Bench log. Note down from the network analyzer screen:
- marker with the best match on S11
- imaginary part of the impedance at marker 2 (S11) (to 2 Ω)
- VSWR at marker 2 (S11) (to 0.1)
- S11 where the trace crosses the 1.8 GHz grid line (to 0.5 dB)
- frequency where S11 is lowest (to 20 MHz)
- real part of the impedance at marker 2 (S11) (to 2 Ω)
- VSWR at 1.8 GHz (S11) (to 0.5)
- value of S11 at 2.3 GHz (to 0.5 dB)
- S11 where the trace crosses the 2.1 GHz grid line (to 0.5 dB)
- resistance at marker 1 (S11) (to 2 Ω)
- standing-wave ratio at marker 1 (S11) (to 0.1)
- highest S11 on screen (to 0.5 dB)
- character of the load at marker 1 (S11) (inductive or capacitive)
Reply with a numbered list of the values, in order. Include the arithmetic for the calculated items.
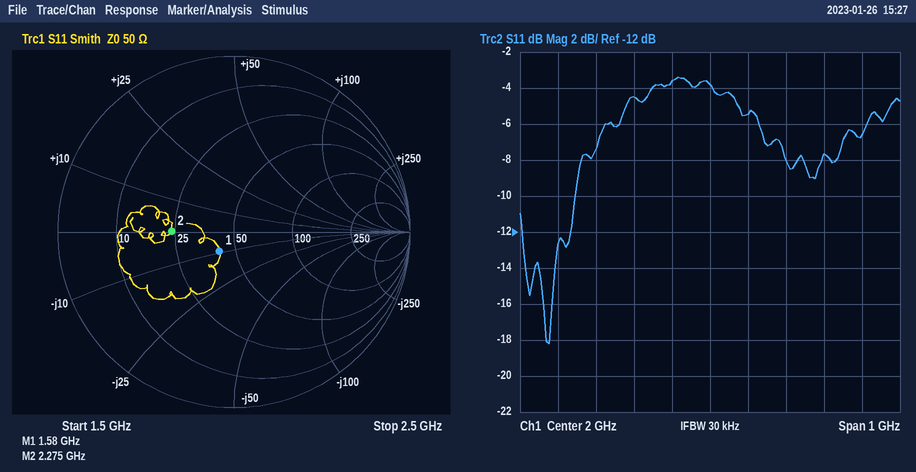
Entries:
1. marker 1
2. 0 Ω
3. 2.1
4. -4.5 dB
5. 1.58 GHz
6. 24 Ω
7. |Γ| = 10^(-4.5/20) = 0.5957; VSWR = (1 + 0.5957)/(1 − 0.5957) ≈ 4.0
8. -7.5 dB
9. -5.5 dB
10. 42 Ω
11. 1.3
12. -3.5 dB
13. capacitive
